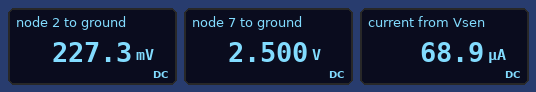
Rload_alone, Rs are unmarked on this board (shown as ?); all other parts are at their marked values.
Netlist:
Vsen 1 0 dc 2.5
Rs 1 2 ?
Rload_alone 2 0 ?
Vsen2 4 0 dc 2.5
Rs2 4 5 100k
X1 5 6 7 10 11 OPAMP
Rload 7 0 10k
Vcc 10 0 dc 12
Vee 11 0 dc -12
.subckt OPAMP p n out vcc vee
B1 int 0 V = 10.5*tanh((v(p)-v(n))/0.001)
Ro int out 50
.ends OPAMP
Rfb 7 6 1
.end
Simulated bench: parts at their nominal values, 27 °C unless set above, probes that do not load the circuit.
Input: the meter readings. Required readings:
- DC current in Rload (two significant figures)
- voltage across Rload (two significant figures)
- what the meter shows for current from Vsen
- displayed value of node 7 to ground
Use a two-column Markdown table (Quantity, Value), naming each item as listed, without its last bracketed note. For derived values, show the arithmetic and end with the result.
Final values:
| Quantity | Value |
|---|---|
| DC current in Rload | (2.5 V) / 10 kΩ = 250 µA |
| voltage across Rload | 2.5 V = 2.5 V |
| what the meter shows for current from Vsen | 68.9 µA |
| displayed value of node 7 to ground | 2.500 V |
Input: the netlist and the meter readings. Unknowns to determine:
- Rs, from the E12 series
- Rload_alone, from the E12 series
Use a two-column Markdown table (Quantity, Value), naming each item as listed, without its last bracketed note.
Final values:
| Quantity | Value |
|---|---|
| Rs, from the E12 series | 33 kΩ |
| Rload_alone, from the E12 series | 3.3 kΩ |
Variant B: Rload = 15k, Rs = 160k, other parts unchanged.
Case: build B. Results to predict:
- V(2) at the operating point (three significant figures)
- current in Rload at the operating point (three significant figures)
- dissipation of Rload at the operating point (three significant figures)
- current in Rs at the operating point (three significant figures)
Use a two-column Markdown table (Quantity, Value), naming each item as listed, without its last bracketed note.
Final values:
| Quantity | Value |
|---|---|
| V(2) at the operating point | 50.5 mV |
| current in Rload at the operating point | 167 µA |
| dissipation of Rload at the operating point | 417 µW |
| current in Rs at the operating point | 15.3 µA |
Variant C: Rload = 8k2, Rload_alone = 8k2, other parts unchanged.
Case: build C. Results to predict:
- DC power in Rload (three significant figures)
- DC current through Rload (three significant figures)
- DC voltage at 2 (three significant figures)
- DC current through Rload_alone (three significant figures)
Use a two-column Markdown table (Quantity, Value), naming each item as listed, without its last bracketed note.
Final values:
| Quantity | Value |
|---|---|
| DC power in Rload | 762 µW |
| DC current through Rload | 305 µA |
| DC voltage at 2 | 498 mV |
| DC current through Rload_alone | 60.7 µA |
